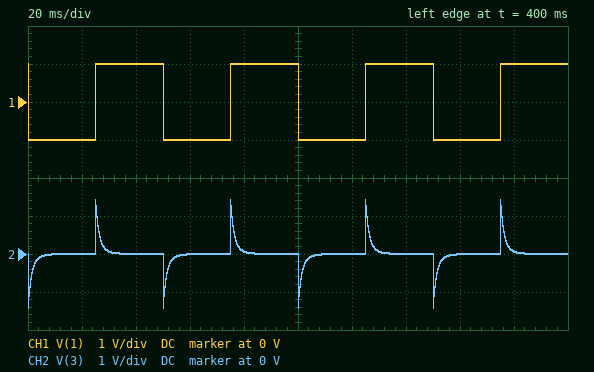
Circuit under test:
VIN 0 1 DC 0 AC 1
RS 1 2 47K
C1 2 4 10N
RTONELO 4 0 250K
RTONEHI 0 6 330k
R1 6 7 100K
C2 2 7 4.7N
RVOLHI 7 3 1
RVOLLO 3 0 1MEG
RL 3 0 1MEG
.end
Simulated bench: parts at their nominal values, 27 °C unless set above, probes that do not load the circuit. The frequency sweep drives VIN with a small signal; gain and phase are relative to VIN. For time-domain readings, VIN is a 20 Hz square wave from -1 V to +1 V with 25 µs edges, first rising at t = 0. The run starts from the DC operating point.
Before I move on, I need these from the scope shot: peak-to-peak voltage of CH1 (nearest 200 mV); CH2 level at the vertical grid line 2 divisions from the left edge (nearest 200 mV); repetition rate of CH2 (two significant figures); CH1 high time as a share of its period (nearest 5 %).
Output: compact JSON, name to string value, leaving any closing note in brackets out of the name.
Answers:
{"peak-to-peak voltage of CH1": "2.0 V", "CH2 level at the vertical grid line 2 divisions from the left edge": "0 V", "repetition rate of CH2": "20 Hz", "CH1 high time as a share of its period": "50 %"}
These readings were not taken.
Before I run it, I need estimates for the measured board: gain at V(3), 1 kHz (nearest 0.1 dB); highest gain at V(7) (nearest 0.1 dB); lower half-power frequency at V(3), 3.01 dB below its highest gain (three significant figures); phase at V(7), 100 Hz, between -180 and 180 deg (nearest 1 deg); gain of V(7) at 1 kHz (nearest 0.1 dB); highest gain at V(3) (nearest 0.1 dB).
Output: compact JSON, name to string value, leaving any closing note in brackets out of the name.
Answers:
{"gain at V(3), 1 kHz": "-2.9 dB", "highest gain at V(7)": "-2.9 dB", "lower half-power frequency at V(3), 3.01 dB below its highest gain": "119 Hz", "phase at V(7), 100 Hz, between -180 and 180 deg": "-133 deg", "gain of V(7) at 1 kHz": "-2.9 dB", "highest gain at V(3)": "-2.9 dB"}
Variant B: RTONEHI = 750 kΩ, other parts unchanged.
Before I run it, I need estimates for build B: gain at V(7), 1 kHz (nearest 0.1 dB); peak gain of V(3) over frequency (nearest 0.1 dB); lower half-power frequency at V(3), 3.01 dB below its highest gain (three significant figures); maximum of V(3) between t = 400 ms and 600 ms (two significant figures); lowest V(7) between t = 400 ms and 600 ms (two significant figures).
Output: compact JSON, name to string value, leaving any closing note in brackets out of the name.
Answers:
{"gain at V(7), 1 kHz": "-2.6 dB", "peak gain of V(3) over frequency": "-2.5 dB", "lower half-power frequency at V(3), 3.01 dB below its highest gain": "87.5 Hz", "maximum of V(3) between t = 400 ms and 600 ms": "1.5 V", "lowest V(7) between t = 400 ms and 600 ms": "-1.5 V"}
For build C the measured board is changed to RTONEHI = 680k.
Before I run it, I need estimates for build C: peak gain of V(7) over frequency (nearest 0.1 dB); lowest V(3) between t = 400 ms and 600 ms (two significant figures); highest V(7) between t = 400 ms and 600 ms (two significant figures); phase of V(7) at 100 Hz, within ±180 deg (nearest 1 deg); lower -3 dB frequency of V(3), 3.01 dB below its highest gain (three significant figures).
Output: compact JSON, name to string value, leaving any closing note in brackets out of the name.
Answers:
{"peak gain of V(7) over frequency": "-2.6 dB", "lowest V(3) between t = 400 ms and 600 ms": "-1.5 V", "highest V(7) between t = 400 ms and 600 ms": "1.5 V", "phase of V(7) at 100 Hz, within ±180 deg": "-140 deg", "lower -3 dB frequency of V(3), 3.01 dB below its highest gain": "90.5 Hz"}
